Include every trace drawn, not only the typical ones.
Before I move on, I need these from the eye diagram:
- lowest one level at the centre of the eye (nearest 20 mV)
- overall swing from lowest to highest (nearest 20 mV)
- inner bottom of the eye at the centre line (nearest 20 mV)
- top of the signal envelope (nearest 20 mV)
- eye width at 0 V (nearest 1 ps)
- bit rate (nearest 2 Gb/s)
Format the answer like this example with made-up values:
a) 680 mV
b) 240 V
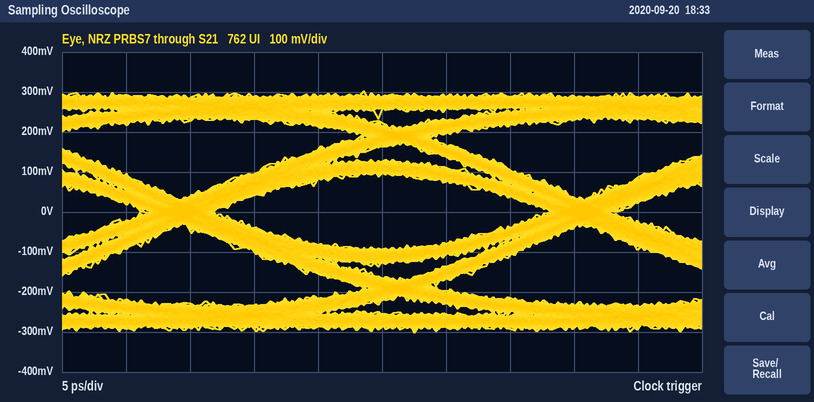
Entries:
a) 100 mV
b) 600 mV
c) -100 mV
d) 300 mV
e) 26 ps
f) 32 Gb/s
